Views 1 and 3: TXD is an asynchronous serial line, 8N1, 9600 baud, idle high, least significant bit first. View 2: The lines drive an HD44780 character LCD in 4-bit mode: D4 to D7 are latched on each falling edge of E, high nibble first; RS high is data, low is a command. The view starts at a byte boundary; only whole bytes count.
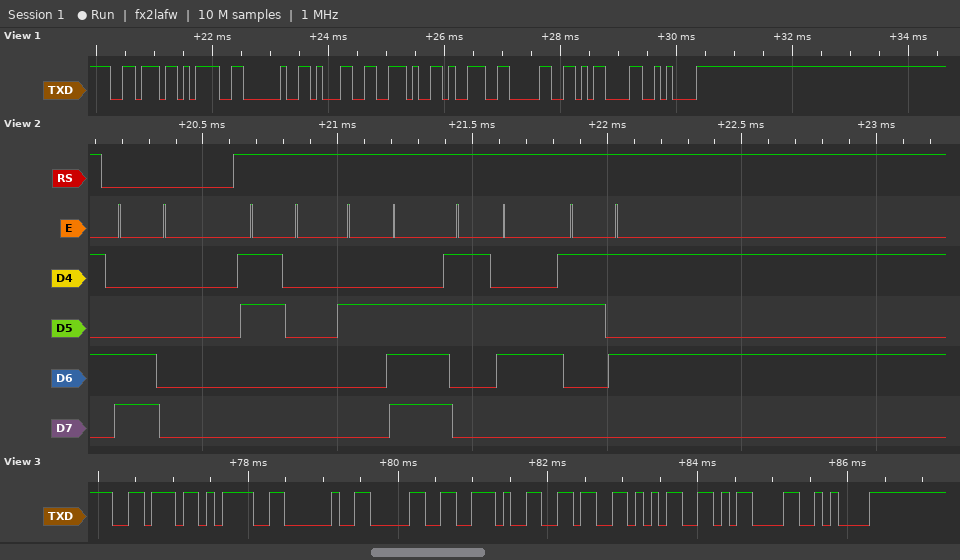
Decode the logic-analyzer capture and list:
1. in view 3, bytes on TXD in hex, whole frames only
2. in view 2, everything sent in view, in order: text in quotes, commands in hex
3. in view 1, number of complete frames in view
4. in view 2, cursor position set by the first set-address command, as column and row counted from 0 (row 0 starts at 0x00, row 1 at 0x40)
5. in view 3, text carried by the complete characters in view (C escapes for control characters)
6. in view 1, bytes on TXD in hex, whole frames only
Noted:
76 3D 20 30 2E 36 35 0D 0A
0xC0 "0.65"
9
column 0, row 1
"v= 0.65\r\n"
76 3D 20 31 2E 39 30 0D 0A
